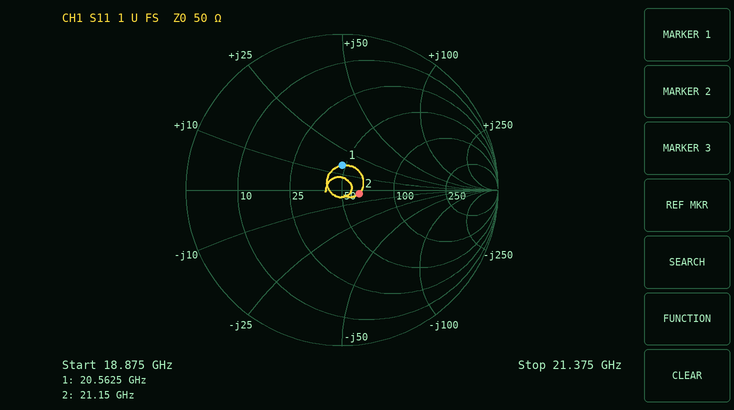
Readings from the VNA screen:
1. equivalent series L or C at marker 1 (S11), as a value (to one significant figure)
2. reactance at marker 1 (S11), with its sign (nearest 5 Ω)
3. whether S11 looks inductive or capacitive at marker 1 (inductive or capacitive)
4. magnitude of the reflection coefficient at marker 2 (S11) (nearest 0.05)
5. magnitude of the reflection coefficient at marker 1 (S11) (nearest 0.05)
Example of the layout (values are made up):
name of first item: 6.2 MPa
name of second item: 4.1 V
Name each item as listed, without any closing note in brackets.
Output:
equivalent series L or C at marker 1 (S11), as a value: 100 pH
reactance at marker 1 (S11), with its sign: +15 Ω
whether S11 looks inductive or capacitive at marker 1: inductive
magnitude of the reflection coefficient at marker 2 (S11): 0.10
magnitude of the reflection coefficient at marker 1 (S11): 0.15
